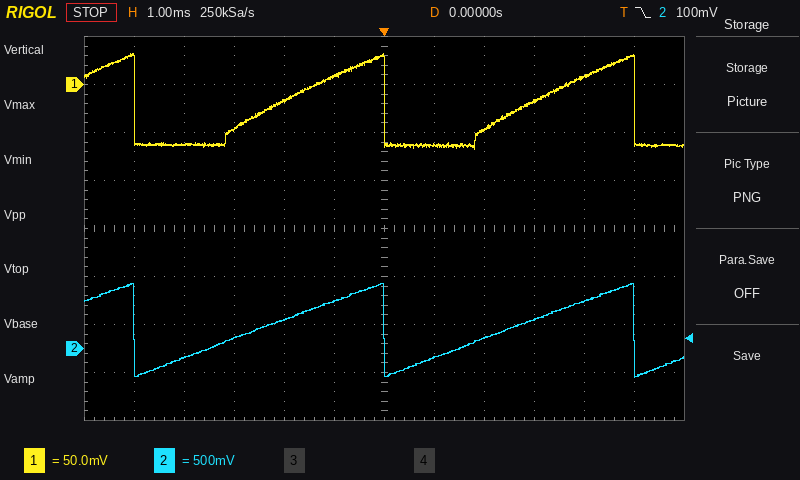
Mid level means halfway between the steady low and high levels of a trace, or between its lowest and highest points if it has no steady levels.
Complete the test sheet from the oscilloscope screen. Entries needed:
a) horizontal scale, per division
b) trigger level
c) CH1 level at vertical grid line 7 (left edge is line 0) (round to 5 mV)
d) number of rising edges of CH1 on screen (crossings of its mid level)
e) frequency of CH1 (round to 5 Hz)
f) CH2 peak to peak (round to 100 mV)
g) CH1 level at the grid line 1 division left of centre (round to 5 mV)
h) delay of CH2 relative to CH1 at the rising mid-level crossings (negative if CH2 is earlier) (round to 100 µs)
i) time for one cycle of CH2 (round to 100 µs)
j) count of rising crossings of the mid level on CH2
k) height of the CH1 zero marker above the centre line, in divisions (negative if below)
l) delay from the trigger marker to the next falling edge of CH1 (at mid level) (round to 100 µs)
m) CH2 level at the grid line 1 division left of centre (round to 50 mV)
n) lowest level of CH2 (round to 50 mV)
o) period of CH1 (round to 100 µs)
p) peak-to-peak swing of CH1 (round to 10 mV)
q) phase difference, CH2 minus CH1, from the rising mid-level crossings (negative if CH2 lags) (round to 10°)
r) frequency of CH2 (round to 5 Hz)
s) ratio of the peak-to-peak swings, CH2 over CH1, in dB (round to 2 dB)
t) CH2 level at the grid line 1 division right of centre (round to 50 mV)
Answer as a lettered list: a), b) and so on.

a) 1 ms
b) 100 mV
c) -65 mV
d) 2
e) 200 Hz
f) 1.00 V
g) 10 mV
h) -600 µs
i) 5.0 ms
j) 2
k) +3.0 div
l) 5.0 ms
m) 500 mV
n) -300 mV
o) 5.0 ms
p) 100 mV
q) +40°
r) 200 Hz
s) 20 dB
t) -100 mV
